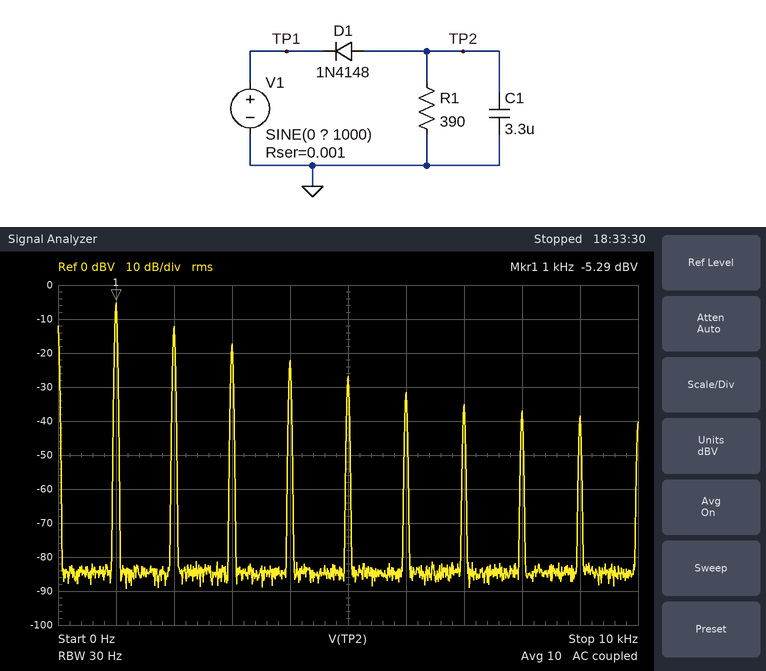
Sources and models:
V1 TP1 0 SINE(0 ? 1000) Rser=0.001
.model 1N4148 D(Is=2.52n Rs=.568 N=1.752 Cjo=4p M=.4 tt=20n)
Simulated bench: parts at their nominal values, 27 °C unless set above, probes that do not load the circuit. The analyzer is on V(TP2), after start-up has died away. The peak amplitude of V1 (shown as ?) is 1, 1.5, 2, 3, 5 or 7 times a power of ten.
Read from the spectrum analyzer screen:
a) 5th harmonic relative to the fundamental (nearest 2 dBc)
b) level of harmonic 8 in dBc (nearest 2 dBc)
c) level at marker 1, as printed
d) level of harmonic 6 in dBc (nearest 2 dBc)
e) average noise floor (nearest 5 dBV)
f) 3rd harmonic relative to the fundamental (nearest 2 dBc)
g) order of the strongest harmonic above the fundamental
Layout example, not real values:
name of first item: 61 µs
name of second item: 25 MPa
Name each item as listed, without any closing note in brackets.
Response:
5th harmonic relative to the fundamental: -22 dBc
level of harmonic 8 in dBc: -32 dBc
level at marker 1, as printed: -5.29 dBV
level of harmonic 6 in dBc: -26 dBc
average noise floor: -85 dBV
3rd harmonic relative to the fundamental: -12 dBc
order of the strongest harmonic above the fundamental: 2
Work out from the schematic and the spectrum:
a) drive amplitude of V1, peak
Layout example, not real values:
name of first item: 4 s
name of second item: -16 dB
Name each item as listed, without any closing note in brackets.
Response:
drive amplitude of V1, peak: 5 V
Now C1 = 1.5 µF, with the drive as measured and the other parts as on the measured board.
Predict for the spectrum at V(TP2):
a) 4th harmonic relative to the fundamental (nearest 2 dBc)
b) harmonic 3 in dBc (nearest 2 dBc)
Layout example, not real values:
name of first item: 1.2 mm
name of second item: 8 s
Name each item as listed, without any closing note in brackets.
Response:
4th harmonic relative to the fundamental: -20 dBc
harmonic 3 in dBc: -14 dBc
